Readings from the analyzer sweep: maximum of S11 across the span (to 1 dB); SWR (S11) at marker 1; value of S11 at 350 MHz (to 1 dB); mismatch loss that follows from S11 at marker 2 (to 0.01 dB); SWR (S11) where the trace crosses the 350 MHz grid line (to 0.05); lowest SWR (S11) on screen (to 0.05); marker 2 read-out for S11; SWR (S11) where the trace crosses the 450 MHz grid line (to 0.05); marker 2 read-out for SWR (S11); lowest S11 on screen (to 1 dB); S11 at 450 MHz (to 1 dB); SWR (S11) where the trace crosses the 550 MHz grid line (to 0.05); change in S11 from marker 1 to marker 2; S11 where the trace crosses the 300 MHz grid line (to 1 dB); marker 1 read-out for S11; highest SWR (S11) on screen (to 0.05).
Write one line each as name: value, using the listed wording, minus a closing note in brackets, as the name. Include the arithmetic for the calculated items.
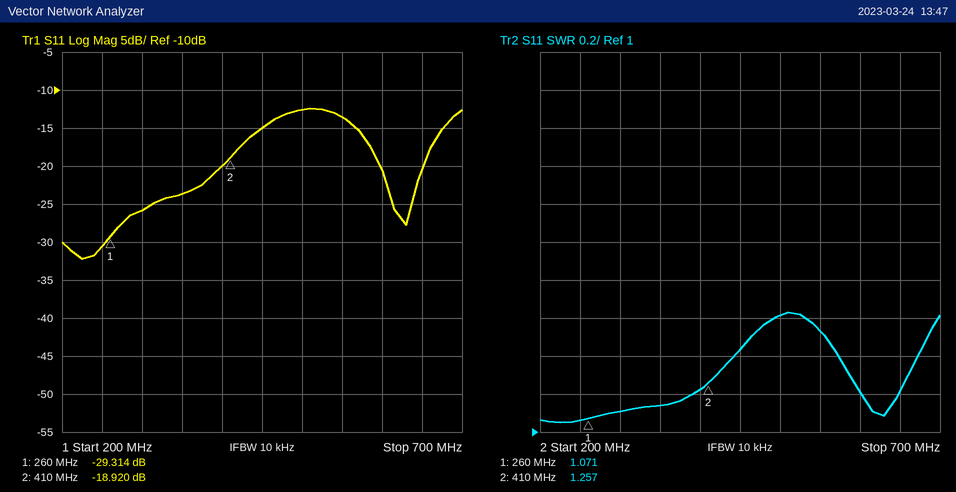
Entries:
maximum of S11 across the span: -12 dB
SWR (S11) at marker 1: 1.071
value of S11 at 350 MHz: -24 dB
mismatch loss that follows from S11 at marker 2: −10 log10(1 − 10^(-18.92/10)) ≈ 0.06 dB
SWR (S11) where the trace crosses the 350 MHz grid line: 1.15
lowest SWR (S11) on screen: 1.05
marker 2 read-out for S11: -18.920 dB
SWR (S11) where the trace crosses the 450 MHz grid line: 1.45
marker 2 read-out for SWR: 1.257
lowest S11 on screen: -32 dB
S11 at 450 MHz: -15 dB
SWR (S11) where the trace crosses the 550 MHz grid line: 1.55
change in S11 from marker 1 to marker 2: -18.92 − (-29.314) = 10.394 dB
S11 where the trace crosses the 300 MHz grid line: -26 dB
marker 1 read-out for S11: -29.314 dB
highest SWR (S11) on screen: 1.65
